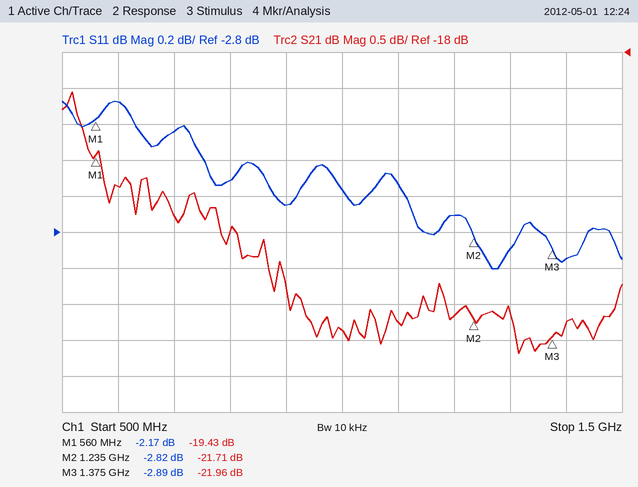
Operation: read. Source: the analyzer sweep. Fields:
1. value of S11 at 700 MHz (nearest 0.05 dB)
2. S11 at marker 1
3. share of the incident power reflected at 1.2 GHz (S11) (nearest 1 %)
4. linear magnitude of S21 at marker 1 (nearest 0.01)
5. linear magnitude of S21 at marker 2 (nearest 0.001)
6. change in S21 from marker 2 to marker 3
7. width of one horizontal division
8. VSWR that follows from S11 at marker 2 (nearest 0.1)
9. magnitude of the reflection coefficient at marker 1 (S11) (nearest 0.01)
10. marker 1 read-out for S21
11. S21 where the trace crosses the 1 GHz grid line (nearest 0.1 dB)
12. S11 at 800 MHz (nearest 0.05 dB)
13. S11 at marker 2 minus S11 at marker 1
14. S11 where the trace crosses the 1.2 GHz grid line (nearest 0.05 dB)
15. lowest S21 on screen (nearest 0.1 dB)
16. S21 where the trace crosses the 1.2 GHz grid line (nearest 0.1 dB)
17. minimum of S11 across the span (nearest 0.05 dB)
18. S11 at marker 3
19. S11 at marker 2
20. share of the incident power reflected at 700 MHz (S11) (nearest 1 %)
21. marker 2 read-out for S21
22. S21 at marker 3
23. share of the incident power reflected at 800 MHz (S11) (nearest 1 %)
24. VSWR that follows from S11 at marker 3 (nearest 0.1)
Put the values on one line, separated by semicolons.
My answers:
-2.25 dB; -2.17 dB; 54 %; 0.11; 0.082; -0.25 dB; 100 MHz; 6.2; 0.78; -19.43 dB; -21.9 dB; -2.50 dB; -0.65 dB; -2.70 dB; -22.2 dB; -21.7 dB; -3.00 dB; -2.89 dB; -2.82 dB; 60 %; -21.71 dB; -21.96 dB; 56 %; 6.1
